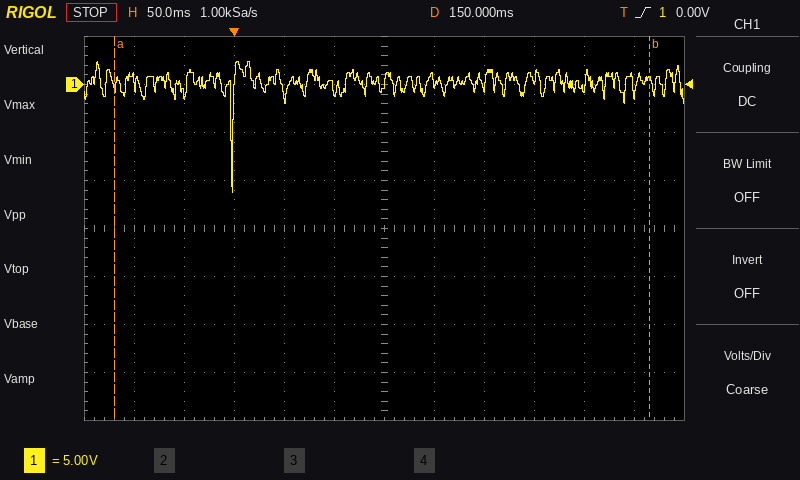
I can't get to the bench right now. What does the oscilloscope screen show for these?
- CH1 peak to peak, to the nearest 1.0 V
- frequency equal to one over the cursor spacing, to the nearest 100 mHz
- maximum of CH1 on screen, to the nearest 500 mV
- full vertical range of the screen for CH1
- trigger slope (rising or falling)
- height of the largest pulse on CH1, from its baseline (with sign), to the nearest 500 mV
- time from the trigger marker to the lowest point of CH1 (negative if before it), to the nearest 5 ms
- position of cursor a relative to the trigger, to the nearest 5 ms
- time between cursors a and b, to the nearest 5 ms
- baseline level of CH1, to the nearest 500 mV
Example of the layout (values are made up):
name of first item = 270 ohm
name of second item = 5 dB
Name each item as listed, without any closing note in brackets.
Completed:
CH1 peak to peak, to the nearest 1.0 V = 14.0 V
frequency equal to one over the cursor spacing, to the nearest 100 mHz = 1.9 Hz
maximum of CH1 on screen, to the nearest 500 mV = 2.5 V
full vertical range of the screen for CH1 = 40 V
trigger slope = rising
height of the largest pulse on CH1, from its baseline (with sign), to the nearest 500 mV = -11.5 V
time from the trigger marker to the lowest point of CH1 (negative if before it), to the nearest 5 ms = 0 ms
position of cursor a relative to the trigger, to the nearest 5 ms = -120 ms
time between cursors a and b, to the nearest 5 ms = 535 ms
baseline level of CH1, to the nearest 500 mV = 500 mV
